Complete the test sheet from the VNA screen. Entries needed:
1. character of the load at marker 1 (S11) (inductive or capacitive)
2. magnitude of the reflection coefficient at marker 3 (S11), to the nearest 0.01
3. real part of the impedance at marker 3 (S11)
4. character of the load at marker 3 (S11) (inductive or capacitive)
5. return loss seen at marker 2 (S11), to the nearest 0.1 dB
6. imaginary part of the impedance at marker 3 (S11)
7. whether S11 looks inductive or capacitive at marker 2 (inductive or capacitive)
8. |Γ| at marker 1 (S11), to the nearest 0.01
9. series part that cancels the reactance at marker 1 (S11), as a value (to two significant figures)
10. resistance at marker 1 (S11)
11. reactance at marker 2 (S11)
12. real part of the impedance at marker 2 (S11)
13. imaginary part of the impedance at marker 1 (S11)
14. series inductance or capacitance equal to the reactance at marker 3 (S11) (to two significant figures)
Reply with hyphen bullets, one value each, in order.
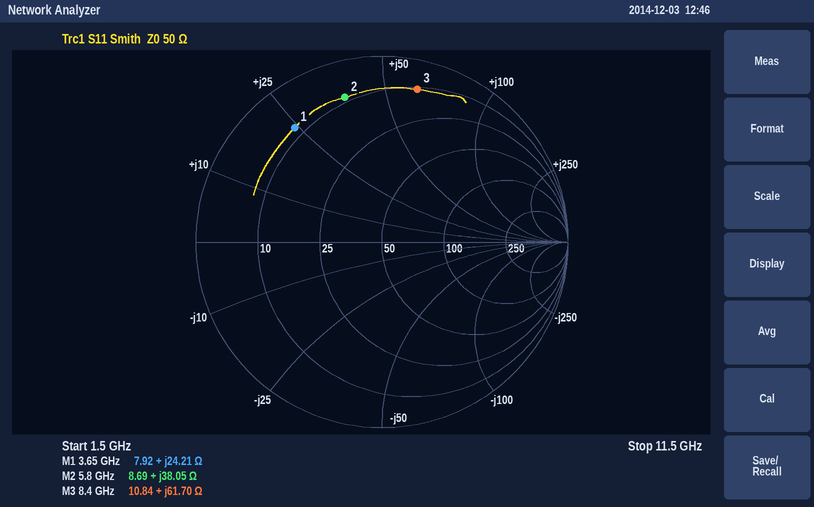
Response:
- inductive
- 0.84
- 10.84 Ω
- inductive
- 1.9 dB
- +61.70 Ω
- inductive
- 0.77
- 1.8 pF
- 7.92 Ω
- +38.05 Ω
- 8.69 Ω
- +24.21 Ω
- 1.2 nH
